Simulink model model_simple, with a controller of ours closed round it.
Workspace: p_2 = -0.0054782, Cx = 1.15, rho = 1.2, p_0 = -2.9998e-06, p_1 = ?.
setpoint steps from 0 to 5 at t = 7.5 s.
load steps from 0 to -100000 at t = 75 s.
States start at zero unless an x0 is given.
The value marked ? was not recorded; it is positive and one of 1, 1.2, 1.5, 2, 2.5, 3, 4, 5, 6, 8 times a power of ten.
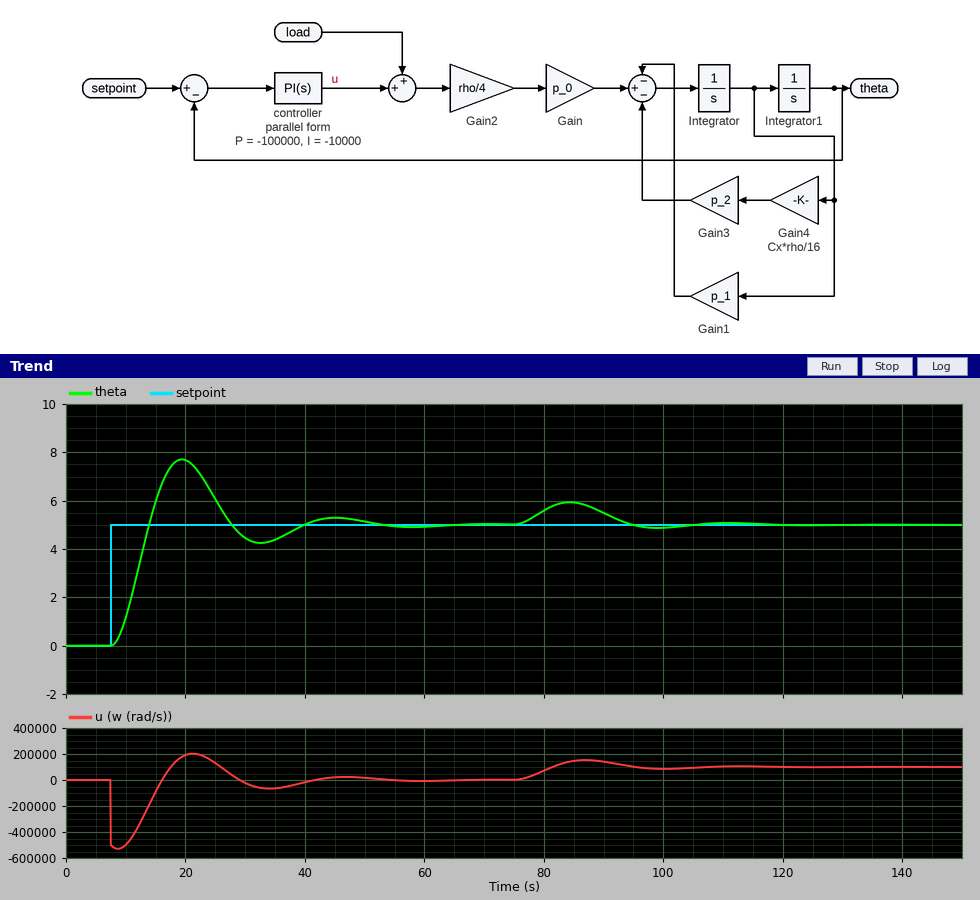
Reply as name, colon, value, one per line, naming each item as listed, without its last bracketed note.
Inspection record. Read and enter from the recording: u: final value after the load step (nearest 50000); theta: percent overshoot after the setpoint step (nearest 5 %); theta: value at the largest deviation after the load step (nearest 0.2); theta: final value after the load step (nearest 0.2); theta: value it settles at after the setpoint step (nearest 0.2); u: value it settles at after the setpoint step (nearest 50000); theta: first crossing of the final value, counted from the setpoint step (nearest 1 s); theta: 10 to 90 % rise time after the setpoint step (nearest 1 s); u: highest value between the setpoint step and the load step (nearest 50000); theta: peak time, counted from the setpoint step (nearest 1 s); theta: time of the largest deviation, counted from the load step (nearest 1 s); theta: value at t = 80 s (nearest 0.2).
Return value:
u: final value after the load step: 100000
theta: percent overshoot after the setpoint step: 55 %
theta: value at the largest deviation after the load step: 6.0
theta: final value after the load step: 5.0
theta: value it settles at after the setpoint step: 5.0
u: value it settles at after the setpoint step: 0
theta: first crossing of the final value, counted from the setpoint step: 6 s
theta: 10 to 90 % rise time after the setpoint step: 4 s
u: highest value between the setpoint step and the load step: 200000
theta: peak time, counted from the setpoint step: 12 s
theta: time of the largest deviation, counted from the load step: 9 s
theta: value at t = 80 s: 5.6
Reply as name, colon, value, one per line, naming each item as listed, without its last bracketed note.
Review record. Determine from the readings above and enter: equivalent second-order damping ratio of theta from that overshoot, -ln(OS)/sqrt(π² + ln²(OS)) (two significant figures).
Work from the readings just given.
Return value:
equivalent second-order damping ratio of theta from that overshoot, -ln(OS)/sqrt(π² + ln²(OS)): 0.19
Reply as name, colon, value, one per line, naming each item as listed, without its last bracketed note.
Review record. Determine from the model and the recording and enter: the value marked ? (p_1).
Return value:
the value marked ?: 0.3
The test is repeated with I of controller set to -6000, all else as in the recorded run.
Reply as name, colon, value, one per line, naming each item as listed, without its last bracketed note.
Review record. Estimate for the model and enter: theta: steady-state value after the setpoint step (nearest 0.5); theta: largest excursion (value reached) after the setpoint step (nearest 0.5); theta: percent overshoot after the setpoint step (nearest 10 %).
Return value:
theta: steady-state value after the setpoint step: 5.0
theta: largest excursion (value reached) after the setpoint step: 7.0
theta: percent overshoot after the setpoint step: 40 %
